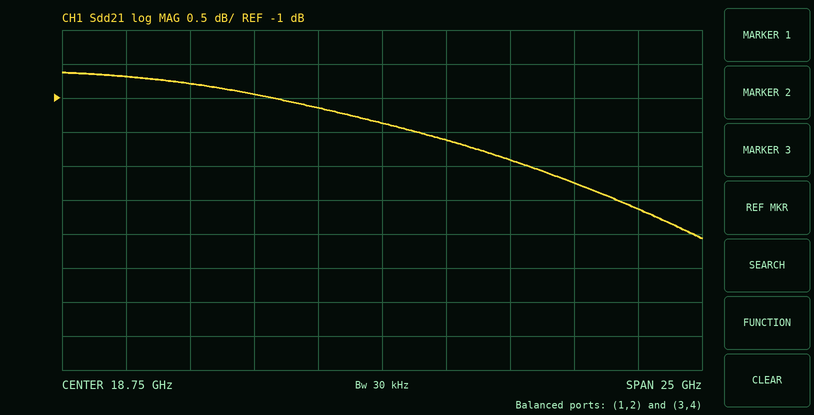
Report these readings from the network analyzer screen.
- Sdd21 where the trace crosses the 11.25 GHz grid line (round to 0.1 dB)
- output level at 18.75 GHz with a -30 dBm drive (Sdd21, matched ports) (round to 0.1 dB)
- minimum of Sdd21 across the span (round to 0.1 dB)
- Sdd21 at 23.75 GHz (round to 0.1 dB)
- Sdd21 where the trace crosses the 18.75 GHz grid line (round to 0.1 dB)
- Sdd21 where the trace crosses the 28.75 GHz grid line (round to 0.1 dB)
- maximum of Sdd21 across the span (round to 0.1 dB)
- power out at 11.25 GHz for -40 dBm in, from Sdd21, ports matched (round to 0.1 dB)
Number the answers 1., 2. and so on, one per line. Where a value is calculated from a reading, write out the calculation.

1. -0.8 dB
2. -30 dBm + (-1.4 dB) = -31.4 dBm
3. -3.1 dB
4. -1.9 dB
5. -1.4 dB
6. -2.6 dB
7. -0.6 dB
8. -40 dBm + (-0.8 dB) = -40.8 dBm
